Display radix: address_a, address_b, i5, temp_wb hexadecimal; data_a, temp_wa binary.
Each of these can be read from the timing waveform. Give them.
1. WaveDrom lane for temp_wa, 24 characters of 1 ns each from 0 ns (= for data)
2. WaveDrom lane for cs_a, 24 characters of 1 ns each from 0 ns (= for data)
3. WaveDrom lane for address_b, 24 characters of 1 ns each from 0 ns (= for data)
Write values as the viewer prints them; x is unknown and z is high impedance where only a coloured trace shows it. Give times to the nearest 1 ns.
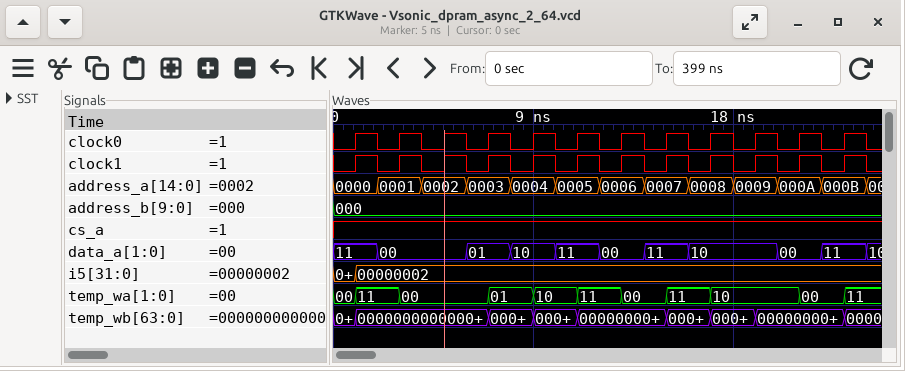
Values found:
{name: 'temp_wa', wave: '==.=...=.=.=.=.=.=...=.=', data: '00 11 00 01 10 11 00 11 10 00 11'}
{name: 'cs_a', wave: '1.......................'}
{name: 'address_b', wave: '=.......................', data: '000'}
